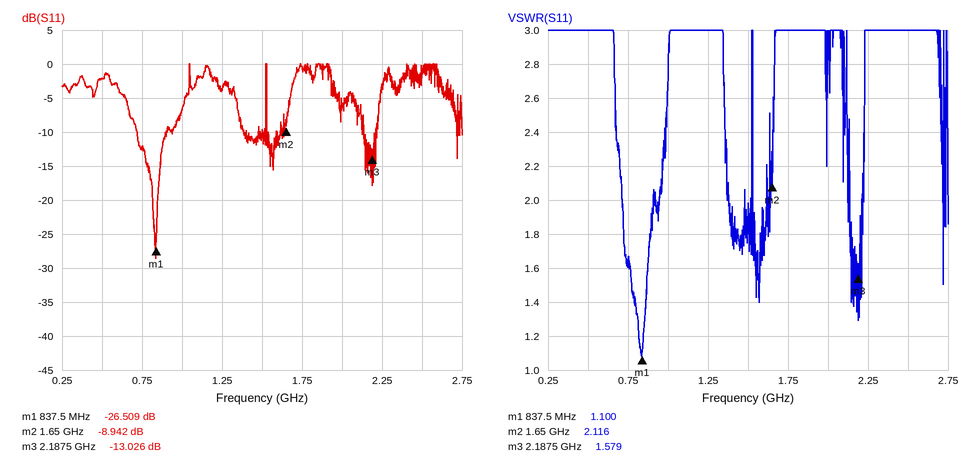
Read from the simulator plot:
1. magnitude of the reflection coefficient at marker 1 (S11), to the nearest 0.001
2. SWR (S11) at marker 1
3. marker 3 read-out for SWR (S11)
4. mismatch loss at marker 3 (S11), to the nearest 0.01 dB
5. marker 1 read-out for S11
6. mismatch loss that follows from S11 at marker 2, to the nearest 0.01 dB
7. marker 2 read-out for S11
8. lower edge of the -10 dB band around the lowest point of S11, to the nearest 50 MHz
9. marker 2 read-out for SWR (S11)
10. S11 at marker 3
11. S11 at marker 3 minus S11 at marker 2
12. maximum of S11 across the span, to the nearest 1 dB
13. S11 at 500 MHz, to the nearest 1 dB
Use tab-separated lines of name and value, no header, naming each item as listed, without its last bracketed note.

magnitude of the reflection coefficient at marker 1 (S11), to the nearest 0.001	0.047
SWR (S11) at marker 1	1.100
marker 3 read-out for SWR	1.579
mismatch loss at marker 3 (S11), to the nearest 0.01 dB	0.22 dB
marker 1 read-out for S11	-26.509 dB
mismatch loss that follows from S11 at marker 2, to the nearest 0.01 dB	0.59 dB
marker 2 read-out for S11	-8.942 dB
lower edge of the -10 dB band around the lowest point of S11, to the nearest 50 MHz	700 MHz
marker 2 read-out for SWR	2.116
S11 at marker 3	-13.026 dB
S11 at marker 3 minus S11 at marker 2	-4.084 dB
maximum of S11 across the span, to the nearest 1 dB	0 dB
S11 at 500 MHz, to the nearest 1 dB	-2 dB
